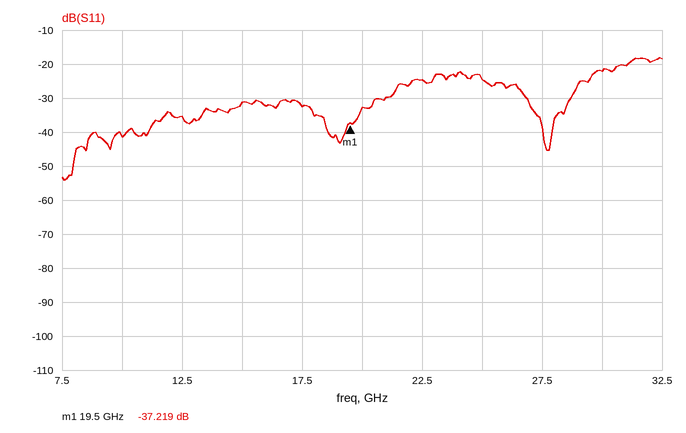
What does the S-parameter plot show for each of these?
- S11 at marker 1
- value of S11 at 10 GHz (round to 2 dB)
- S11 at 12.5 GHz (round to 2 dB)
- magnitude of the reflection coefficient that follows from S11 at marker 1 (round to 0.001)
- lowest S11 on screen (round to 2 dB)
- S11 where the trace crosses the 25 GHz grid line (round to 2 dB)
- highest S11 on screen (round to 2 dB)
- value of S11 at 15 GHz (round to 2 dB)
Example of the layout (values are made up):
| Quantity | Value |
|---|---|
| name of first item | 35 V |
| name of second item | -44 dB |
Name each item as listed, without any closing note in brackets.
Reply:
| Quantity | Value |
|---|---|
| S11 at marker 1 | -37.219 dB |
| value of S11 at 10 GHz | -42 dB |
| S11 at 12.5 GHz | -36 dB |
| magnitude of the reflection coefficient that follows from S11 at marker 1 | 0.014 |
| lowest S11 on screen | -54 dB |
| S11 where the trace crosses the 25 GHz grid line | -24 dB |
| highest S11 on screen | -18 dB |
| value of S11 at 15 GHz | -32 dB |
